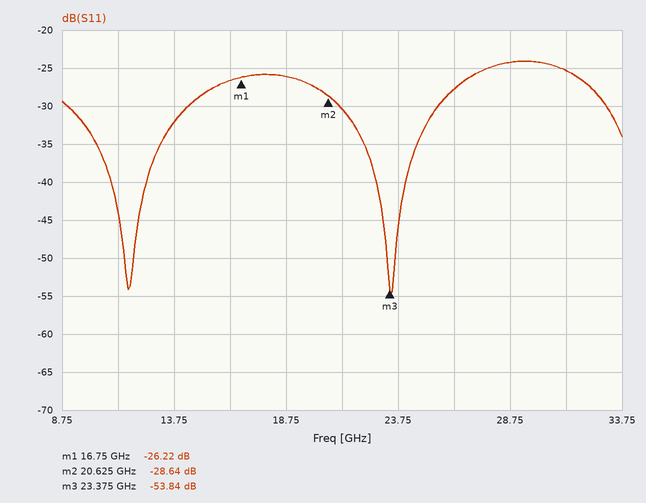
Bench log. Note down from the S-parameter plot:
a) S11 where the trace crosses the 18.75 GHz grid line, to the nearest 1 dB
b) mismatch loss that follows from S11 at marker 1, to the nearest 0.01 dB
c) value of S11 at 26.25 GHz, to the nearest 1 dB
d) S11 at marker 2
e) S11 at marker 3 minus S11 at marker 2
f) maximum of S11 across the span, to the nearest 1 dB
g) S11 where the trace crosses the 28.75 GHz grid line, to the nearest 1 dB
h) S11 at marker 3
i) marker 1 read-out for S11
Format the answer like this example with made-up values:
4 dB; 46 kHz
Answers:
-26 dB; 0.01 dB; -28 dB; -28.64 dB; -25.20 dB; -24 dB; -24 dB; -53.84 dB; -26.22 dB
